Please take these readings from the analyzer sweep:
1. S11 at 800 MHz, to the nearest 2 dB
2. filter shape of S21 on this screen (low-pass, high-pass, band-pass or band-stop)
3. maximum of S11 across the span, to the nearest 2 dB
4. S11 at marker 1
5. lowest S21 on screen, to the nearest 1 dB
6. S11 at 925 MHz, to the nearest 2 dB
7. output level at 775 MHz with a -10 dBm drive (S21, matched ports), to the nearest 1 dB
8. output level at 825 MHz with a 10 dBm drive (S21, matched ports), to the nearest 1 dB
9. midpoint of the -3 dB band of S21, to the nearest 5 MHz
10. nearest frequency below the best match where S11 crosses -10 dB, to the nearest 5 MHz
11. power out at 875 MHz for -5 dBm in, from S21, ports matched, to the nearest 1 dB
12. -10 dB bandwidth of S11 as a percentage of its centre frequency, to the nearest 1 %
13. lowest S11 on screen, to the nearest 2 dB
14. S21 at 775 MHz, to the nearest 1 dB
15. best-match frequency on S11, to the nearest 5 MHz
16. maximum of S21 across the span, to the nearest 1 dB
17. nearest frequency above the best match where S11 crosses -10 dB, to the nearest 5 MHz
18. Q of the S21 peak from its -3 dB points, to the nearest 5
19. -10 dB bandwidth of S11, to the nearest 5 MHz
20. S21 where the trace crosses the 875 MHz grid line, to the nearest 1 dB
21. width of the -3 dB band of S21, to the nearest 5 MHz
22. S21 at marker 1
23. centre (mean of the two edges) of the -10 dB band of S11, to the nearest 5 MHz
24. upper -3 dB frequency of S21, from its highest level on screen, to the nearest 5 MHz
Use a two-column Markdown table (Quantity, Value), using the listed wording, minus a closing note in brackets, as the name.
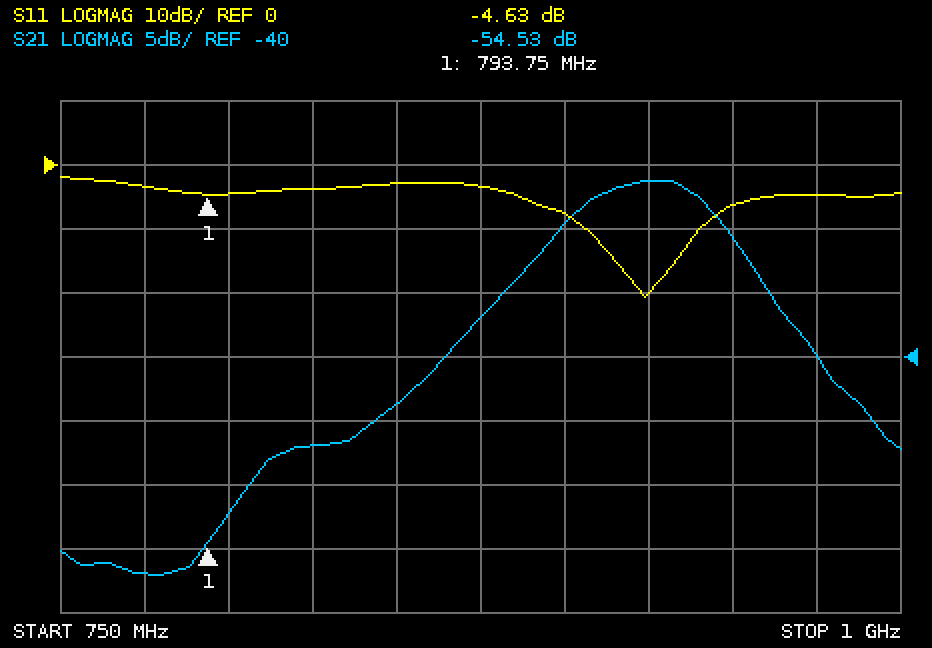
| Quantity | Value |
|---|---|
| S11 at 800 MHz, to the nearest 2 dB | -4 dB |
| filter shape of S21 on this screen | band-pass |
| maximum of S11 across the span, to the nearest 2 dB | -2 dB |
| S11 at marker 1 | -4.63 dB |
| lowest S21 on screen, to the nearest 1 dB | -57 dB |
| S11 at 925 MHz, to the nearest 2 dB | -20 dB |
| output level at 775 MHz with a -10 dBm drive (S21, matched ports), to the nearest 1 dB | -67 dBm |
| output level at 825 MHz with a 10 dBm drive (S21, matched ports), to the nearest 1 dB | -37 dBm |
| midpoint of the -3 dB band of S21, to the nearest 5 MHz | 925 MHz |
| nearest frequency below the best match where S11 crosses -10 dB, to the nearest 5 MHz | 905 MHz |
| power out at 875 MHz for -5 dBm in, from S21, ports matched, to the nearest 1 dB | -42 dBm |
| -10 dB bandwidth of S11 as a percentage of its centre frequency, to the nearest 1 % | 4 % |
| lowest S11 on screen, to the nearest 2 dB | -20 dB |
| S21 at 775 MHz, to the nearest 1 dB | -57 dB |
| best-match frequency on S11, to the nearest 5 MHz | 925 MHz |
| maximum of S21 across the span, to the nearest 1 dB | -26 dB |
| nearest frequency above the best match where S11 crosses -10 dB, to the nearest 5 MHz | 940 MHz |
| Q of the S21 peak from its -3 dB points, to the nearest 5 | 20 |
| -10 dB bandwidth of S11, to the nearest 5 MHz | 35 MHz |
| S21 where the trace crosses the 875 MHz grid line, to the nearest 1 dB | -37 dB |
| width of the -3 dB band of S21, to the nearest 5 MHz | 45 MHz |
| S21 at marker 1 | -54.53 dB |
| centre (mean of the two edges) of the -10 dB band of S11, to the nearest 5 MHz | 925 MHz |
| upper -3 dB frequency of S21, from its highest level on screen, to the nearest 5 MHz | 945 MHz |
